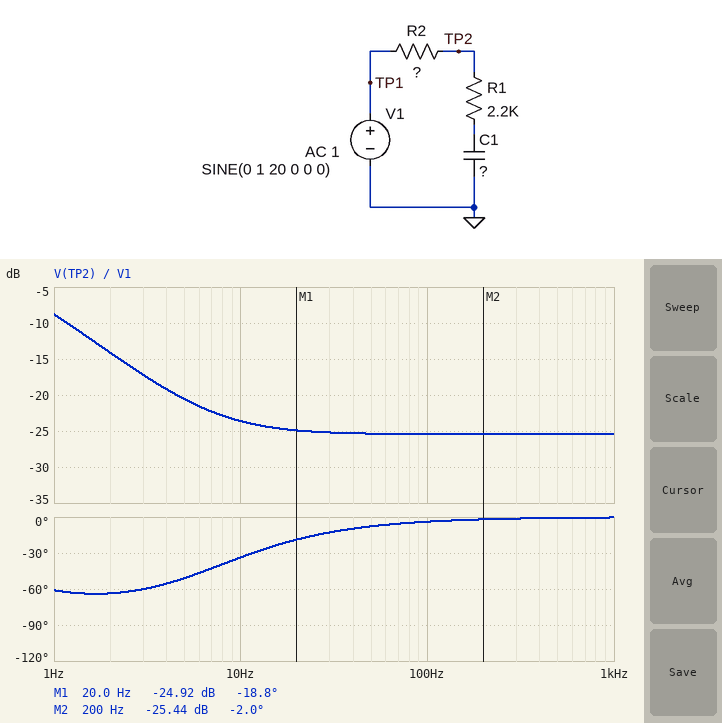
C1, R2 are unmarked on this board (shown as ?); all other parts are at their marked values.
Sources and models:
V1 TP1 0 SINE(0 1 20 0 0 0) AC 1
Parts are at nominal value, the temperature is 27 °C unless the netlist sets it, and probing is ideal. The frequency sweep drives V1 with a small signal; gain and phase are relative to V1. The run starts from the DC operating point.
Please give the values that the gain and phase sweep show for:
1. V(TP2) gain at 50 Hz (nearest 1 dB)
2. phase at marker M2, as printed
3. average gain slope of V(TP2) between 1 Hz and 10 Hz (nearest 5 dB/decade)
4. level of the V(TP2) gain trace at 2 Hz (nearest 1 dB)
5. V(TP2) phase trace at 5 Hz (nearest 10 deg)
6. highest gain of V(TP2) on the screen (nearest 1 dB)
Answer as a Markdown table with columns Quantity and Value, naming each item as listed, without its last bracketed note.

| Quantity | Value |
|---|---|
| V(TP2) gain at 50 Hz | -25 dB |
| phase at marker M2, as printed | -2.0 deg |
| average gain slope of V(TP2) between 1 Hz and 10 Hz | -15 dB/decade |
| level of the V(TP2) gain trace at 2 Hz | -14 dB |
| V(TP2) phase trace at 5 Hz | -50 deg |
| highest gain of V(TP2) on the screen | -9 dB |
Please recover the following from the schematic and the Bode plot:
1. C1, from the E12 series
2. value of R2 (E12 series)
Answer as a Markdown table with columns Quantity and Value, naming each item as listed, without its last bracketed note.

| Quantity | Value |
|---|---|
| C1, from the E12 series | 10 µF |
| value of R2 | 39 kΩ |
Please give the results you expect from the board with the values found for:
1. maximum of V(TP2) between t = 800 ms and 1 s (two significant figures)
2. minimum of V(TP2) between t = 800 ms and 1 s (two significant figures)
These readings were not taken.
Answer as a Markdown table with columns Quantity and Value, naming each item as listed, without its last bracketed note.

| Quantity | Value |
|---|---|
| maximum of V(TP2) between t = 800 ms and 1 s | 59 mV |
| minimum of V(TP2) between t = 800 ms and 1 s | -55 mV |
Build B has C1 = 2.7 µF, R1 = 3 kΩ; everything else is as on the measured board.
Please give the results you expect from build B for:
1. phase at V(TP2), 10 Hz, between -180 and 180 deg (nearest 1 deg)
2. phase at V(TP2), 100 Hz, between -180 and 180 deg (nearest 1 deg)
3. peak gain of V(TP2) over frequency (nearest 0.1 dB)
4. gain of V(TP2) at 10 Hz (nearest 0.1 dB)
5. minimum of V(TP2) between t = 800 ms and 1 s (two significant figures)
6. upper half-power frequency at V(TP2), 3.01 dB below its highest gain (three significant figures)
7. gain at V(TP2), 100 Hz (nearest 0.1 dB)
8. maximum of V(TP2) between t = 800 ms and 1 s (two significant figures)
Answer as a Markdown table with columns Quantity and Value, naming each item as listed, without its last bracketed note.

| Quantity | Value |
|---|---|
| phase at V(TP2), 10 Hz, between -180 and 180 deg | -55 deg |
| phase at V(TP2), 100 Hz, between -180 and 180 deg | -10 deg |
| peak gain of V(TP2) over frequency | 0 dB |
| gain of V(TP2) at 10 Hz | -16.1 dB |
| minimum of V(TP2) between t = 800 ms and 1 s | -100 mV |
| upper half-power frequency at V(TP2), 3.01 dB below its highest gain | 1.41 Hz |
| gain at V(TP2), 100 Hz | -22.8 dB |
| maximum of V(TP2) between t = 800 ms and 1 s | 100 mV |
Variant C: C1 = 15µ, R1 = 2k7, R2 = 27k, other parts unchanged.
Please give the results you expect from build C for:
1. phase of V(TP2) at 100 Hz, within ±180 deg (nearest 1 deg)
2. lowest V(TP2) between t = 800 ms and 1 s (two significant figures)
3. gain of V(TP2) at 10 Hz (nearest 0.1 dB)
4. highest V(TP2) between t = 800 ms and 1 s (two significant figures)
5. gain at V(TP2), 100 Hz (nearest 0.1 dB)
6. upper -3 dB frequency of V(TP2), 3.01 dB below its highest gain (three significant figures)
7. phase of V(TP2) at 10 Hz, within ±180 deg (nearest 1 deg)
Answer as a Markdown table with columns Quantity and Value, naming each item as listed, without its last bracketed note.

| Quantity | Value |
|---|---|
| phase of V(TP2) at 100 Hz, within ±180 deg | -2 deg |
| lowest V(TP2) between t = 800 ms and 1 s | -91 mV |
| gain of V(TP2) at 10 Hz | -20.2 dB |
| highest V(TP2) between t = 800 ms and 1 s | 95 mV |
| gain at V(TP2), 100 Hz | -20.8 dB |
| upper -3 dB frequency of V(TP2), 3.01 dB below its highest gain | 360 mHz |
| phase of V(TP2) at 10 Hz, within ±180 deg | -19 deg |
